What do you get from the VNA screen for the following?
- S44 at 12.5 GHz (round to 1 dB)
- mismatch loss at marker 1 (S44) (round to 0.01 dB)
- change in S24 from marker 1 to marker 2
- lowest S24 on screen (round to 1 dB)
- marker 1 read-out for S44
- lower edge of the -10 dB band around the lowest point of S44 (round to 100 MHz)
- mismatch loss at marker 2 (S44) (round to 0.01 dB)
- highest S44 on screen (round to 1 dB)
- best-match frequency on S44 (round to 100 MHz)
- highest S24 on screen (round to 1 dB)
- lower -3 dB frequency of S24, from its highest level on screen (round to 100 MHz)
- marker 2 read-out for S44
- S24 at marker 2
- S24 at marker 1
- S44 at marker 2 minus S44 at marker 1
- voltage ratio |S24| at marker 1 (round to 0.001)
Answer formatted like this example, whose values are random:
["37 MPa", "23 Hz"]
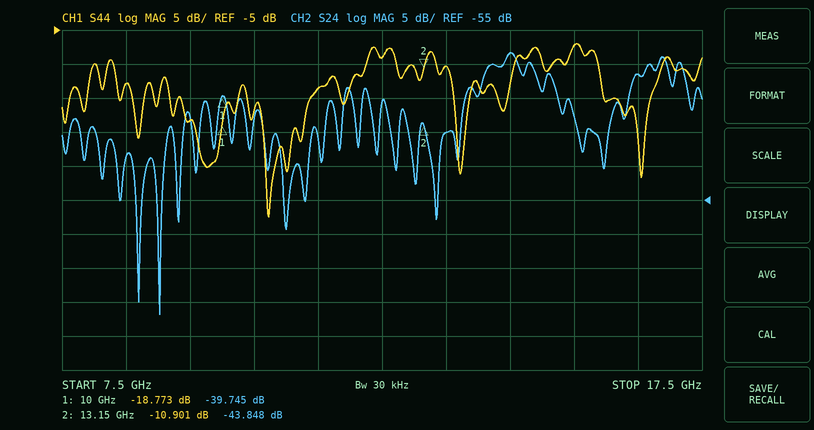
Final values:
["-9 dB", "0.06 dB", "-4.103 dB", "-72 dB", "-18.773 dB", "8.3 GHz", "0.37 dB", "-7 dB", "10.7 GHz", "-33 dB", "14.1 GHz", "-10.901 dB", "-43.848 dB", "-39.745 dB", "7.872 dB", "0.010"]
